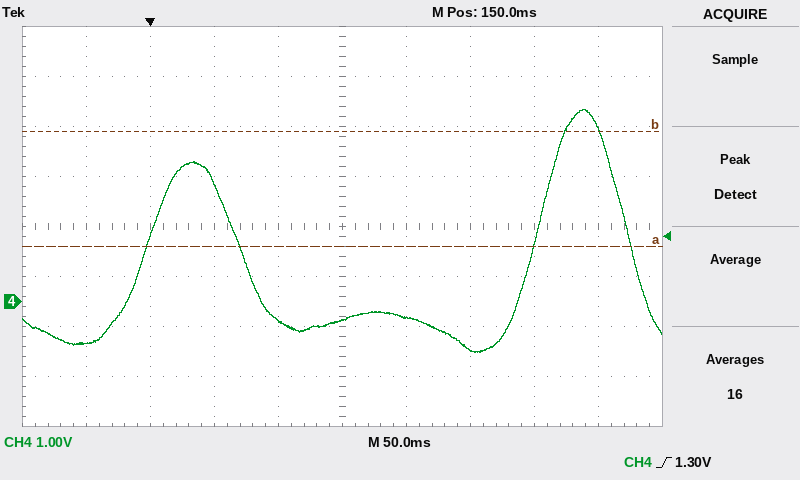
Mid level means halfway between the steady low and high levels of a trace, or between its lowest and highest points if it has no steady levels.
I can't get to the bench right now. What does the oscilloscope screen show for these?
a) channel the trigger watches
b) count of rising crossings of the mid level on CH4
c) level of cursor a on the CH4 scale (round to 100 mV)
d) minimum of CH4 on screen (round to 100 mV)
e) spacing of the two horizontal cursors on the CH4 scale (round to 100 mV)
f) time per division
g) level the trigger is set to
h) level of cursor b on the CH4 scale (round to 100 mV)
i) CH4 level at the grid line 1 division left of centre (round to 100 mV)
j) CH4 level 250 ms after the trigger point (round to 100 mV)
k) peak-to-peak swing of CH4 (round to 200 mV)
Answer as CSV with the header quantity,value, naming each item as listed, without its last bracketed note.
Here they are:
quantity,value
channel the trigger watches,CH4
count of rising crossings of the mid level on CH4,2
level of cursor a on the CH4 scale,1.1 V
minimum of CH4 on screen,-1.0 V
spacing of the two horizontal cursors on the CH4 scale,2.3 V
time per division,50 ms
level the trigger is set to,1.30 V
level of cursor b on the CH4 scale,3.4 V
CH4 level at the grid line 1 division left of centre,-400 mV
CH4 level 250 ms after the trigger point,-1.0 V
peak-to-peak swing of CH4,4.8 V
